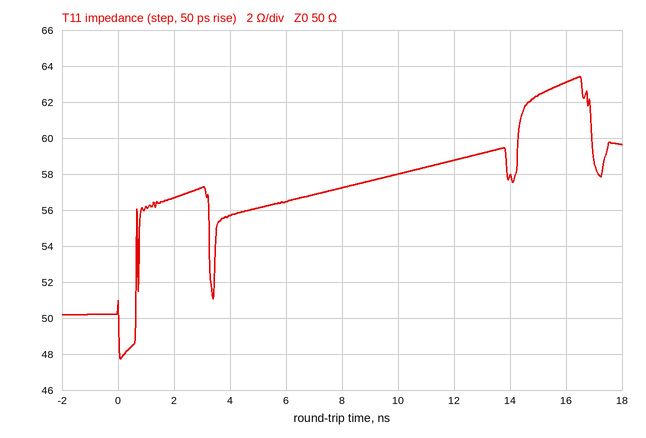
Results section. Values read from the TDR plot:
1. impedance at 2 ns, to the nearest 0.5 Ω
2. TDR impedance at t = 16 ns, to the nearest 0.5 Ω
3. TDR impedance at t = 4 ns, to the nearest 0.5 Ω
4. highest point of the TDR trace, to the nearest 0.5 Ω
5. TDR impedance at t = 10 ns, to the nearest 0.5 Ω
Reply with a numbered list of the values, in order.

1. 56.5 Ω
2. 63.0 Ω
3. 55.5 Ω
4. 63.5 Ω
5. 58.0 Ω
